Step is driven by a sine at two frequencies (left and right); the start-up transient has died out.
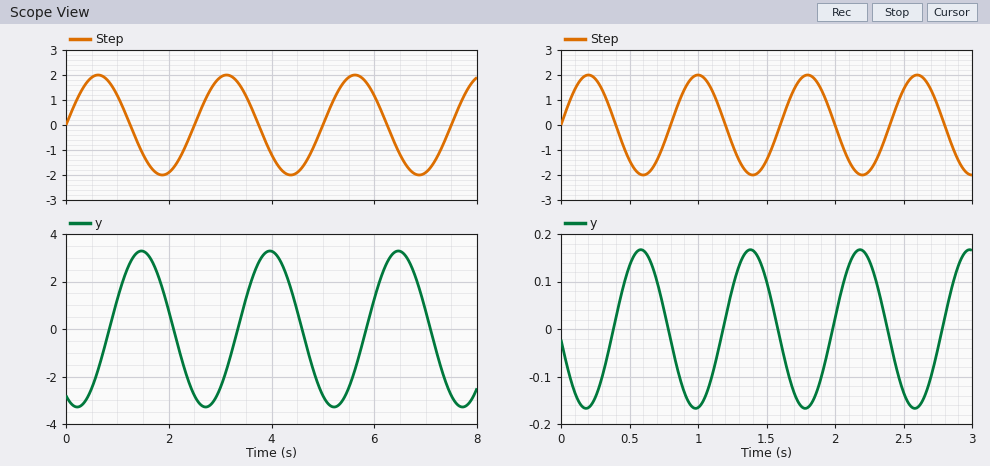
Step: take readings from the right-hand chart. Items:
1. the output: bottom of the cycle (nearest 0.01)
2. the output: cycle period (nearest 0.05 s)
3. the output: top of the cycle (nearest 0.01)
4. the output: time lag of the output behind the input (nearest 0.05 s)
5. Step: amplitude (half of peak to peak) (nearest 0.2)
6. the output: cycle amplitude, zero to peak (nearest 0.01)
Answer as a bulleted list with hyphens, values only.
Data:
- -0.17
- 0.80 s
- 0.17
- 0.40 s
- 2.0
- 0.17
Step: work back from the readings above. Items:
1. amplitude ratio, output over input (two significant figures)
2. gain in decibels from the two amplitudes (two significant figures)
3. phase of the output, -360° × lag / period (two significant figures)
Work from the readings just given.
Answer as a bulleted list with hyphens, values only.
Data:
- 0.085
- -21 dB
- -180°
